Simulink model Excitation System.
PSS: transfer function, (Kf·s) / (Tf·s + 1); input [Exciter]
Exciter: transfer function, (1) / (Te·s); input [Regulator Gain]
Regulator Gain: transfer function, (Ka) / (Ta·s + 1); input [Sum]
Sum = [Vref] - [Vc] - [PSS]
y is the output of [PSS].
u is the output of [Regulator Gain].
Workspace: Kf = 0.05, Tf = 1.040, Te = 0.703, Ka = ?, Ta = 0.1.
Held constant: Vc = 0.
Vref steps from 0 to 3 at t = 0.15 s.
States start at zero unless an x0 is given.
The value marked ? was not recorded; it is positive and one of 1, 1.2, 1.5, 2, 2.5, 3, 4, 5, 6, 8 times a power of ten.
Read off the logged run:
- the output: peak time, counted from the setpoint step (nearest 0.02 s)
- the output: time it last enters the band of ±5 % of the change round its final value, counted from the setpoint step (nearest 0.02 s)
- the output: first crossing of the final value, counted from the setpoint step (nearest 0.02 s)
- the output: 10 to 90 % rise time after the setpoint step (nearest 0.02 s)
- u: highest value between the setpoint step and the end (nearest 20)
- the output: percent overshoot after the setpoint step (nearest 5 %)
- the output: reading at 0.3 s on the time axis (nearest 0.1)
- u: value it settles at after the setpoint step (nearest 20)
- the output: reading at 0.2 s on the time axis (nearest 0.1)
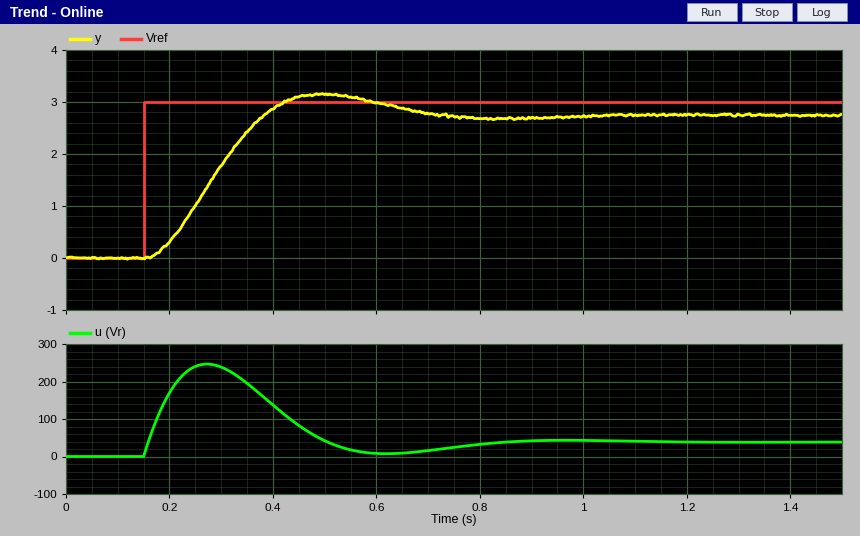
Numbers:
0.34 s
0.50 s
0.24 s
0.16 s
240
15 %
1.8
40
0.3
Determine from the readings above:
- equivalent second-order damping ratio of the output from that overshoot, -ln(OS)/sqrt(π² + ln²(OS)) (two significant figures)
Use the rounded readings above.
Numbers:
0.52
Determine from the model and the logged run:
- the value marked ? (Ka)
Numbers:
150
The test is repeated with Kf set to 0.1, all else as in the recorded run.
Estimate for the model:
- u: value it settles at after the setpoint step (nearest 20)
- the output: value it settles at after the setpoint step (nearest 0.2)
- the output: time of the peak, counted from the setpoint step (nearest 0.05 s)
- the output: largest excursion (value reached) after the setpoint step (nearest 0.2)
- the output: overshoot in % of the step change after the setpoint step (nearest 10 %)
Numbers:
20
2.8
0.25 s
3.6
30 %
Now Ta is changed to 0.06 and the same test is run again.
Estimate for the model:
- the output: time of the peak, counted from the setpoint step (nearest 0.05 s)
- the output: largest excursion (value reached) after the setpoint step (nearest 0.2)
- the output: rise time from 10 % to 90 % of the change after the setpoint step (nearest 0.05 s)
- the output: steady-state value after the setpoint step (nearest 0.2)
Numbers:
0.30 s
3.0
0.15 s
2.8
